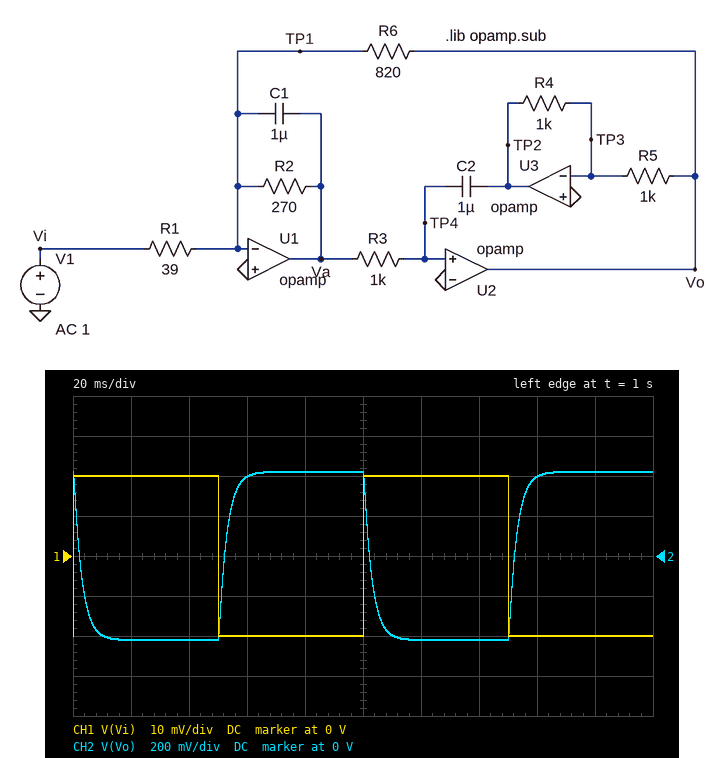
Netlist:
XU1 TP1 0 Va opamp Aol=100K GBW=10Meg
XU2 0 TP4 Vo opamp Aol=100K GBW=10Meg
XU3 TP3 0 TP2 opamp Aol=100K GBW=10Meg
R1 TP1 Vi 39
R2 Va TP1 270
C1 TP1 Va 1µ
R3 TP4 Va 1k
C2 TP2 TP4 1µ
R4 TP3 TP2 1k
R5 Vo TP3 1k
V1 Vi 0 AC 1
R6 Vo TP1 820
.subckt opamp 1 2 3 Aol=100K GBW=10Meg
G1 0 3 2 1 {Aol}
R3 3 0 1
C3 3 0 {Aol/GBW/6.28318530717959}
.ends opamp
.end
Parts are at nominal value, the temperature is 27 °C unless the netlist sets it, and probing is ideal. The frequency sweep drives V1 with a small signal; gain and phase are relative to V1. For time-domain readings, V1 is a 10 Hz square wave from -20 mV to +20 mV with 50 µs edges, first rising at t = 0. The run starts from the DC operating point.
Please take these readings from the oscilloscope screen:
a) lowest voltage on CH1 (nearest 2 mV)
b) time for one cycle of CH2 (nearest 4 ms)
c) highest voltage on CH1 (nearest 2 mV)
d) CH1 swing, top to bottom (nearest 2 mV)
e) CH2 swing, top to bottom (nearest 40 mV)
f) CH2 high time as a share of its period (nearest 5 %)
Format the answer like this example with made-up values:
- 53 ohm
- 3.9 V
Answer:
- -20 mV
- 100 ms
- 20 mV
- 40 mV
- 840 mV
- 50 %
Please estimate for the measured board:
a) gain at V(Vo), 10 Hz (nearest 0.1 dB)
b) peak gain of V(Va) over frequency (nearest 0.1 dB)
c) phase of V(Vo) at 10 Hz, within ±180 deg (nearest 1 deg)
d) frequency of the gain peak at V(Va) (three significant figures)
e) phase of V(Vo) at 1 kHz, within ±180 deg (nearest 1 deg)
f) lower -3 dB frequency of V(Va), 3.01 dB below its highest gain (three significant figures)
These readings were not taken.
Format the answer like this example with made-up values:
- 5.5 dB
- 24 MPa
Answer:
- 26.3 dB
- 16.8 dB
- 169 deg
- 176 Hz
- 31 deg
- 48.4 Hz
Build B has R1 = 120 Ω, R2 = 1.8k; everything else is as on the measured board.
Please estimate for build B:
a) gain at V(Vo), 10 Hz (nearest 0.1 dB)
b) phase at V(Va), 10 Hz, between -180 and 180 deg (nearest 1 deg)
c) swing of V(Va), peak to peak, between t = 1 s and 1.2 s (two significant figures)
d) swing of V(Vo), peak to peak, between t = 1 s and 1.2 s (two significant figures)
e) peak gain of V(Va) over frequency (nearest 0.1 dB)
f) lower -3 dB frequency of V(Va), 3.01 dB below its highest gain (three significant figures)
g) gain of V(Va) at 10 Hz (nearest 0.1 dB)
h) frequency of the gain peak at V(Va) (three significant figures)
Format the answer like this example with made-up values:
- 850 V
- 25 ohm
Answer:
- 16.7 dB
- -92 deg
- 430 mV
- 520 mV
- 23.5 dB
- 137 Hz
- -7.3 dB
- 176 Hz
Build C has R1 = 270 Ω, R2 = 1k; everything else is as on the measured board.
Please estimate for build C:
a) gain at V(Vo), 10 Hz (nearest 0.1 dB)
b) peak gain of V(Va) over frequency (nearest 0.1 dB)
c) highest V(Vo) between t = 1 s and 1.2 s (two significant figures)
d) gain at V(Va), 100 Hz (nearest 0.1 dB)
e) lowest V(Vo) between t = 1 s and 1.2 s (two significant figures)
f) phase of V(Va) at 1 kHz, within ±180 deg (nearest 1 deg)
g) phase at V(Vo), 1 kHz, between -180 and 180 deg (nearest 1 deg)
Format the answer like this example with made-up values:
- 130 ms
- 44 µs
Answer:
- 9.7 dB
- 11.4 dB
- 86 mV
- 7.0 dB
- -86 mV
- 99 deg
- 9 deg
